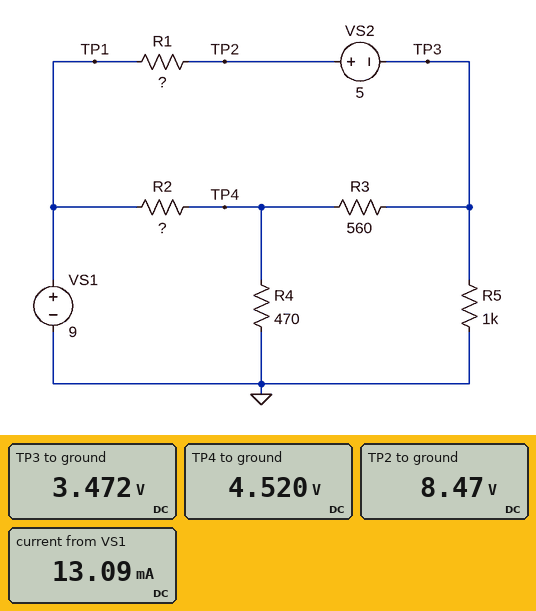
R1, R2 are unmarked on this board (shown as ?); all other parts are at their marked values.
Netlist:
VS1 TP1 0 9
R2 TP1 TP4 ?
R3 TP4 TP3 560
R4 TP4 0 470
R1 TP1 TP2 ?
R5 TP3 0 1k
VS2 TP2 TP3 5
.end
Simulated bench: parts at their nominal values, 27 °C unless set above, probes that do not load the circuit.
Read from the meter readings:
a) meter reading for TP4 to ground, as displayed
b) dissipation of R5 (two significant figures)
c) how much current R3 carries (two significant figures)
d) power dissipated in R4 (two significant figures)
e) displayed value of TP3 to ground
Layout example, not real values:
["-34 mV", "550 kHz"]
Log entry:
["4.520 V", "12 mW", "1.9 mA", "43 mW", "3.472 V"]
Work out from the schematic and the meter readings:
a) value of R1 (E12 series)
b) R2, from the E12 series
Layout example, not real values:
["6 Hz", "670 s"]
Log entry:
["330 Ω", "390 Ω"]
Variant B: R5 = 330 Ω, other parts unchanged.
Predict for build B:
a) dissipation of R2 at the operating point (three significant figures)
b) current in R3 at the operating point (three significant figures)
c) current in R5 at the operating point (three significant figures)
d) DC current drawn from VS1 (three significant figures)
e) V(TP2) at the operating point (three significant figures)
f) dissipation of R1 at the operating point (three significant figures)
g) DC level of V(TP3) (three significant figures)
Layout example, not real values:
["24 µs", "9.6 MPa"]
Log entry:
["57.7 mW", "3.11 mA", "7.62 mA", "16.7 mA", "7.51 V", "6.70 mW", "2.51 V"]
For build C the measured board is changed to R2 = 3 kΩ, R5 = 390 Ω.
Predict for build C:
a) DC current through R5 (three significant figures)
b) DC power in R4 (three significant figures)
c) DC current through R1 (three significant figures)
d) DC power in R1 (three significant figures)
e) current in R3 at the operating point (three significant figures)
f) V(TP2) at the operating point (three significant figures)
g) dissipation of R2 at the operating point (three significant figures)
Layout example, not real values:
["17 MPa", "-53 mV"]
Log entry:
["5.18 mA", "5.15 mW", "6.00 mA", "11.9 mW", "828 µA", "7.02 V", "18.5 mW"]
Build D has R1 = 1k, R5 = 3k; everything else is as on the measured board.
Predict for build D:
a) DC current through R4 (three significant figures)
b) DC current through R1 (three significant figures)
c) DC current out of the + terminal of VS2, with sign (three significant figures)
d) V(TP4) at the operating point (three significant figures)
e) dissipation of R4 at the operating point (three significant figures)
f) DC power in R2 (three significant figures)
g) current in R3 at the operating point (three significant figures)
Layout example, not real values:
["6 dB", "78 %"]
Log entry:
["9.89 mA", "55.3 µA", "-55.3 µA", "4.65 V", "46.0 mW", "48.5 mW", "1.26 mA"]
